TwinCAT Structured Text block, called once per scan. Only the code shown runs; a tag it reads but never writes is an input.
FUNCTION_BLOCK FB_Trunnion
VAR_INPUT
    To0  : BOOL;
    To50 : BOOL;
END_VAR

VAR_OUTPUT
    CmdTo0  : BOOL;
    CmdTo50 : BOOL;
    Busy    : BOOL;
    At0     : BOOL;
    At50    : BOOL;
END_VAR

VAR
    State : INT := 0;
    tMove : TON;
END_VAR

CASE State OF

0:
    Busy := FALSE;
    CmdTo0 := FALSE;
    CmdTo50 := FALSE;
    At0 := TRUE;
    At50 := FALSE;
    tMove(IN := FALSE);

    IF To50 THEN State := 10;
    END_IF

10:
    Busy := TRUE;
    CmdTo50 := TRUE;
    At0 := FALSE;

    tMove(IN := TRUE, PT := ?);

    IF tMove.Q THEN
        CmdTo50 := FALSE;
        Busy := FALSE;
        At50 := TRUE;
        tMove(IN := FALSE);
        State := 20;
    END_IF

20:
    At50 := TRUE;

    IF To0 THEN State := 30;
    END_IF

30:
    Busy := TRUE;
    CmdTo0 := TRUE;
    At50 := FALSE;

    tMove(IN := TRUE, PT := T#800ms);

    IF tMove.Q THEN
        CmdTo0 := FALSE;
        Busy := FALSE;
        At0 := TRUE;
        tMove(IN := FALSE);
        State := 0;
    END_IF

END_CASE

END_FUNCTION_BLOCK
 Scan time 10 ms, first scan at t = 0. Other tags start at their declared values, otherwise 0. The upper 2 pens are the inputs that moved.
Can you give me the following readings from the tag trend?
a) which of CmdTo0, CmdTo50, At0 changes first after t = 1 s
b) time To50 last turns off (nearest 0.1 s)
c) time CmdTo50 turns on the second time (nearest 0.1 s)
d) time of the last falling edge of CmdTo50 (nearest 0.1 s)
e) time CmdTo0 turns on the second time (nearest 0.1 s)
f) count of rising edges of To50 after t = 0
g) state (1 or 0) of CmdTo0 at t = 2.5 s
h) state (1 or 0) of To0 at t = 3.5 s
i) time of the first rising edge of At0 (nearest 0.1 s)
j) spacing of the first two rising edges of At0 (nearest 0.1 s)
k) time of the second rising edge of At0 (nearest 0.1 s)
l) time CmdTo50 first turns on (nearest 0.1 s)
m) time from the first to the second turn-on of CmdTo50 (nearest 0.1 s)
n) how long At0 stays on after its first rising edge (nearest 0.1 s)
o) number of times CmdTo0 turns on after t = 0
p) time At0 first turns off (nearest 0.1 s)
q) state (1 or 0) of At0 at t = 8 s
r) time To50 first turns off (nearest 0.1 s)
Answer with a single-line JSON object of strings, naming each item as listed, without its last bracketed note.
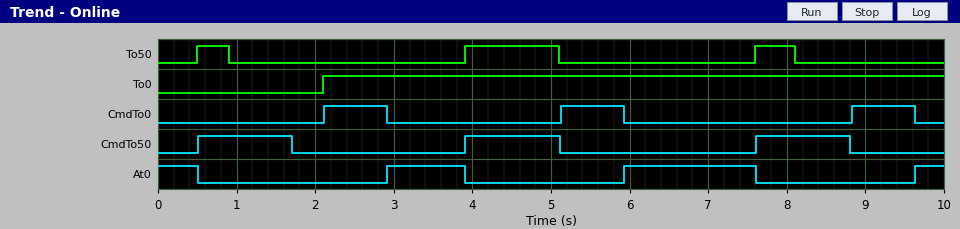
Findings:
{"which of CmdTo0, CmdTo50, At0 changes first after t = 1 s": "CmdTo50", "time To50 last turns off": "8.1 s", "time CmdTo50 turns on the second time": "3.9 s", "time of the last falling edge of CmdTo50": "8.8 s", "time CmdTo0 turns on the second time": "5.1 s", "count of rising edges of To50 after t = 0": "3", "state (1 or 0) of CmdTo0 at t = 2.5 s": "1", "state (1 or 0) of To0 at t = 3.5 s": "1", "time of the first rising edge of At0": "2.9 s", "spacing of the first two rising edges of At0": "3.0 s", "time of the second rising edge of At0": "5.9 s", "time CmdTo50 first turns on": "0.5 s", "time from the first to the second turn-on of CmdTo50": "3.4 s", "how long At0 stays on after its first rising edge": "1.0 s", "number of times CmdTo0 turns on after t = 0": "3", "time At0 first turns off": "0.5 s", "state (1 or 0) of At0 at t = 8 s": "0", "time To50 first turns off": "0.9 s"}
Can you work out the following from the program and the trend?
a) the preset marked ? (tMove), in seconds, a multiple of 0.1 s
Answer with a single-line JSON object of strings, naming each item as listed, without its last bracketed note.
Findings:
{"the preset marked ? (tMove), in seconds, a multiple of 0.1 s": "1.2 s"}
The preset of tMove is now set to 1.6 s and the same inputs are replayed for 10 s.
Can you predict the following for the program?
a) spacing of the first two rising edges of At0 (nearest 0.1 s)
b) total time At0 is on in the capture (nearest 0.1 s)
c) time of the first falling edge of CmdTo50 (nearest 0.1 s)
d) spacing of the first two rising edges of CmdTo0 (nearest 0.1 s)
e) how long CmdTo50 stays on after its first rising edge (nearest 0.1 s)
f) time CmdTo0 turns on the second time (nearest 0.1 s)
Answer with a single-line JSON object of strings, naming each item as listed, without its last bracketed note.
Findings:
{"spacing of the first two rising edges of At0": "3.4 s", "total time At0 is on in the capture": "2.8 s", "time of the first falling edge of CmdTo50": "2.1 s", "spacing of the first two rising edges of CmdTo0": "3.4 s", "how long CmdTo50 stays on after its first rising edge": "1.6 s", "time CmdTo0 turns on the second time": "5.5 s"}
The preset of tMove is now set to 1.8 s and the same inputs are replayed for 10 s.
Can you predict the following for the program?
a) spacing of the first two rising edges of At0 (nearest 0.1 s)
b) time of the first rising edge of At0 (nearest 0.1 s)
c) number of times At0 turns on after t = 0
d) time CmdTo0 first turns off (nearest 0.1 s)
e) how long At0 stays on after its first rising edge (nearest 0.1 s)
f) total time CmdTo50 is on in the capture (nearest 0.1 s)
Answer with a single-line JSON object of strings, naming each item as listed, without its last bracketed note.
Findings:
{"spacing of the first two rising edges of At0": "3.4 s", "time of the first rising edge of At0": "3.1 s", "number of times At0 turns on after t = 0": "2", "time CmdTo0 first turns off": "3.1 s", "how long At0 stays on after its first rising edge": "0.8 s", "total time CmdTo50 is on in the capture": "5.4 s"}
